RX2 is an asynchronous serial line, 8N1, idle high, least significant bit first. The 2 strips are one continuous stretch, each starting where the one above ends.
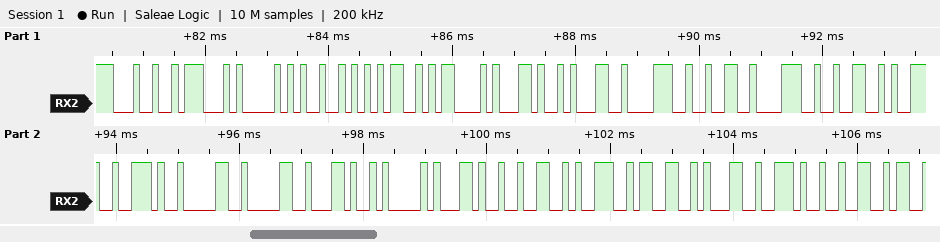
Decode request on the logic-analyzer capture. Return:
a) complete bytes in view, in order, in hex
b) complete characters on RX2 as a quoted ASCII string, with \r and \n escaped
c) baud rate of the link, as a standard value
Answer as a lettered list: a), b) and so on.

a) 24 47 50 52 4D 43 2C 31 38 32 38 32 39 2E 30 30 2C 41 2C 32 39 33 31 2E 32
b) "$GPRMC,182829.00,A,2931.2"
c) 9600 baud
